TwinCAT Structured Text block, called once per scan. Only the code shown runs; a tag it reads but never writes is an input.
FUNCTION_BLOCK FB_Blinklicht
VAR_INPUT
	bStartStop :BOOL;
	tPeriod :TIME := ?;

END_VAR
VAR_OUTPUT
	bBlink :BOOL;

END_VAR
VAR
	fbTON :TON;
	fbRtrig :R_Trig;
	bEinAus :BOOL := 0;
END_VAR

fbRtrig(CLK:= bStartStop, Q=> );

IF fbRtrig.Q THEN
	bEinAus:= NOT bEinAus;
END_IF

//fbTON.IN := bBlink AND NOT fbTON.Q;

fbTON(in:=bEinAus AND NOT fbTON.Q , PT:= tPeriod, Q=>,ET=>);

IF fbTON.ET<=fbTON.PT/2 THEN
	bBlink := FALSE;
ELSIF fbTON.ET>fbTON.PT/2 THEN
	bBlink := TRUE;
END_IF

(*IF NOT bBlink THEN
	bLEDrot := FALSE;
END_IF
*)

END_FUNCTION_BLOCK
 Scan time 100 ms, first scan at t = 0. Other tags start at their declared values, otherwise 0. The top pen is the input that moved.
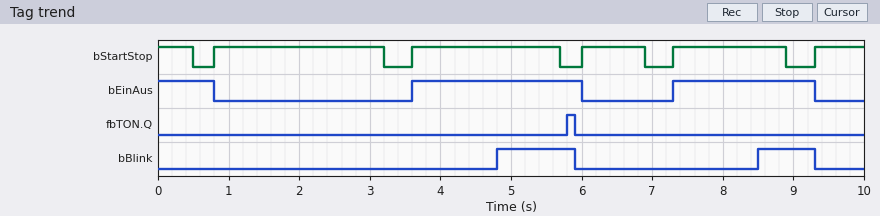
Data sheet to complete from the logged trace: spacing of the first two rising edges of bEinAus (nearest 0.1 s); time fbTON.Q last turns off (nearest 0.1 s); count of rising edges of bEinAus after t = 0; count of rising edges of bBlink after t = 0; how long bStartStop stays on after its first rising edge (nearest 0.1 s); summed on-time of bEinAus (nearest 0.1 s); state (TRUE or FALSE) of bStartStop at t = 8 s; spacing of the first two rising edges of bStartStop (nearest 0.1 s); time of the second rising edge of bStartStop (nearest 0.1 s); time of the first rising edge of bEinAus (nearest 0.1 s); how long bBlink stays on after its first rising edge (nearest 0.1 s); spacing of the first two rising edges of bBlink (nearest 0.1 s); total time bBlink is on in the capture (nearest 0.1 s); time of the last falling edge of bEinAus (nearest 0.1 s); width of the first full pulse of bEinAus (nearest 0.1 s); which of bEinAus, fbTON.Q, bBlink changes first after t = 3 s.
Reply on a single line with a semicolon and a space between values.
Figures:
3.7 s; 5.9 s; 2; 2; 2.4 s; 5.2 s; TRUE; 2.8 s; 3.6 s; 3.6 s; 1.1 s; 3.7 s; 1.9 s; 9.3 s; 2.4 s; bEinAus
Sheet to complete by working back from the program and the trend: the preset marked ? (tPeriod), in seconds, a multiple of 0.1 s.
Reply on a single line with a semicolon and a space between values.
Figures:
2.2 s
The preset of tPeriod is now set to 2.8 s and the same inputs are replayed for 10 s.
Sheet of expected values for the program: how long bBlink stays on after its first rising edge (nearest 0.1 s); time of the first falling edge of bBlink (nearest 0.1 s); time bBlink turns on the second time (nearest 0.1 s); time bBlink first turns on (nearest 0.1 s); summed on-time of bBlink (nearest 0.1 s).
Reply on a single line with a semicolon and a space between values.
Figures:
0.9 s; 6.0 s; 8.8 s; 5.1 s; 1.4 s
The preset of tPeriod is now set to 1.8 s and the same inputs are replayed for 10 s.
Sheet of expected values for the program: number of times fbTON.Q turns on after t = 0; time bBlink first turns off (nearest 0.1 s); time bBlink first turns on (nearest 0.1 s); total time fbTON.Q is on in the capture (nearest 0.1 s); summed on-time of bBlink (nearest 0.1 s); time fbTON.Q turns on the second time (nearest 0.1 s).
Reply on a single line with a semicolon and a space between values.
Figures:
2; 5.5 s; 4.6 s; 0.2 s; 1.8 s; 9.1 s
